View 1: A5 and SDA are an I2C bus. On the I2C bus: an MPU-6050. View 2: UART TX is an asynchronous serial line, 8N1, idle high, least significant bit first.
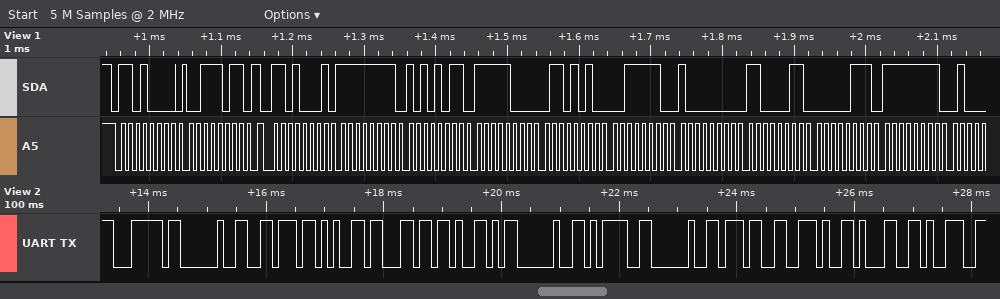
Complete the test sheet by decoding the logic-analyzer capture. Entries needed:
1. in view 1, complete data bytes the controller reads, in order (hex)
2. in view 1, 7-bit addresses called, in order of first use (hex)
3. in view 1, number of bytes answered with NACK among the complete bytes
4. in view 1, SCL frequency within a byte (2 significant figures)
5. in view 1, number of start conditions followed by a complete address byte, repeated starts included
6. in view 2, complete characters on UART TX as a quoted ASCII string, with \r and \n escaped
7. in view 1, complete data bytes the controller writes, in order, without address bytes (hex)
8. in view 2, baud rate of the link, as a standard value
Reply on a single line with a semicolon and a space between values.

FF AB F8 6A 3E 80 C3 07 FF; 0x68; 0; 100 kHz; 2; "| velY = 7.19"; 3B; 9600 baud
